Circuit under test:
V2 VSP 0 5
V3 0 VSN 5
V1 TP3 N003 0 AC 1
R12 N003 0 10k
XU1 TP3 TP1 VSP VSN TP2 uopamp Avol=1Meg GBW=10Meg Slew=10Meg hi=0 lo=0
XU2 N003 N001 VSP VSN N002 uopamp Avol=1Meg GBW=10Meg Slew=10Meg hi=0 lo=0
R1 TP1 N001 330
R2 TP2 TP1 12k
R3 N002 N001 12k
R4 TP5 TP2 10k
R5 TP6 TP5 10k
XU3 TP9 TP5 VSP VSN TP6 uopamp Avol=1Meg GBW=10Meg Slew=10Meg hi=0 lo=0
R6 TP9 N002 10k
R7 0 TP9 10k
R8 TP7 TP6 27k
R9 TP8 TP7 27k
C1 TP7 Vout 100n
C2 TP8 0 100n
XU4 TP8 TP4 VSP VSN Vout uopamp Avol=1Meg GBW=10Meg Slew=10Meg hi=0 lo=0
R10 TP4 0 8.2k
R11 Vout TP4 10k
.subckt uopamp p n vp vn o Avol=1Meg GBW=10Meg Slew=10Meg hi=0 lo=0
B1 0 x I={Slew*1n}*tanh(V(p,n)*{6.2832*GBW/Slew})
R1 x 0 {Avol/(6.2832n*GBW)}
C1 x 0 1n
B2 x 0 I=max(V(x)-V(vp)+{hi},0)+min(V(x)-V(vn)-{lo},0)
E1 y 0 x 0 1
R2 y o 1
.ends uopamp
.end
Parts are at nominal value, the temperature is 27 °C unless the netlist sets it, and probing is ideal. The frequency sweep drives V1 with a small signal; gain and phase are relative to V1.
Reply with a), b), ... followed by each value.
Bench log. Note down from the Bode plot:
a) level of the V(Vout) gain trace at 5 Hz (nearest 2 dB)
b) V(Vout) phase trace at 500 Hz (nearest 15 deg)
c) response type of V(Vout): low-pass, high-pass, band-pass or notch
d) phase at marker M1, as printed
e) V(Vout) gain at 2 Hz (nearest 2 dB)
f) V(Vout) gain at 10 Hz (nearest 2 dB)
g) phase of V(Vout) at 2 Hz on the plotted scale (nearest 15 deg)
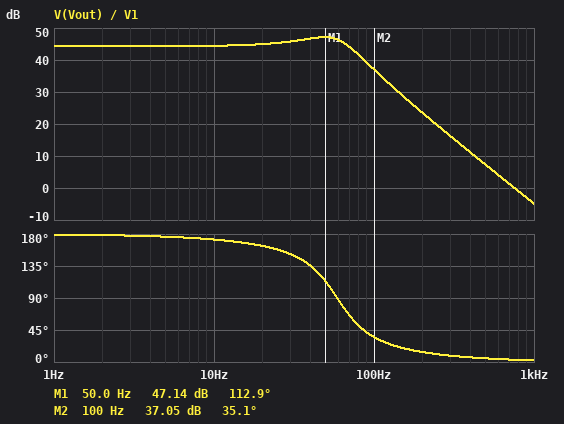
a) 44 dB
b) 0 deg
c) low-pass
d) 112.9 deg
e) 44 dB
f) 44 dB
g) 180 deg
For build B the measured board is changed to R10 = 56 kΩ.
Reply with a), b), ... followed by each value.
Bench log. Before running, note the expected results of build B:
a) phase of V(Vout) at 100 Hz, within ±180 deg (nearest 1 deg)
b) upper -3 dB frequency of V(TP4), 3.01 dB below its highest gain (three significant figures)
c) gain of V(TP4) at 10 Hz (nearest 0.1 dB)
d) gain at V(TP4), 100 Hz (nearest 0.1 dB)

a) 59 deg
b) 43.3 Hz
c) 37.2 dB
d) 26.2 dB
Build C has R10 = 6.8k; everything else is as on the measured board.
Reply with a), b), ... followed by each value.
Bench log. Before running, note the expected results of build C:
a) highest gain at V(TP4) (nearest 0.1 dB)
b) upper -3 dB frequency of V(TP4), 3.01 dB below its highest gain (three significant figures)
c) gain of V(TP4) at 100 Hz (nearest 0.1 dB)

a) 43.2 dB
b) 69.0 Hz
c) 31.0 dB
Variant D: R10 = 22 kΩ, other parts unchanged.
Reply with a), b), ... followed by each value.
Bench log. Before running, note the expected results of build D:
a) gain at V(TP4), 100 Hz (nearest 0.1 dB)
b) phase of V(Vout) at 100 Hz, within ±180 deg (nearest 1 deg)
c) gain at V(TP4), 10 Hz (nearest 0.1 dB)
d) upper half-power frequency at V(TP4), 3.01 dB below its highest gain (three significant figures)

a) 27.2 dB
b) 54 deg
c) 37.3 dB
d) 53.5 Hz
